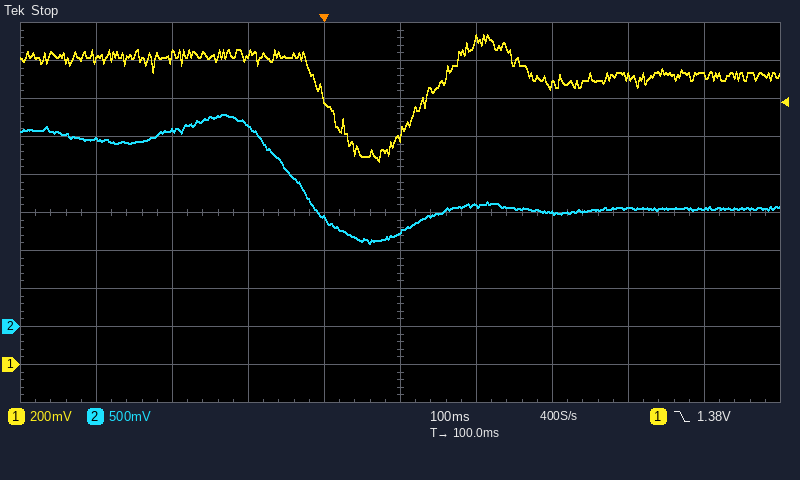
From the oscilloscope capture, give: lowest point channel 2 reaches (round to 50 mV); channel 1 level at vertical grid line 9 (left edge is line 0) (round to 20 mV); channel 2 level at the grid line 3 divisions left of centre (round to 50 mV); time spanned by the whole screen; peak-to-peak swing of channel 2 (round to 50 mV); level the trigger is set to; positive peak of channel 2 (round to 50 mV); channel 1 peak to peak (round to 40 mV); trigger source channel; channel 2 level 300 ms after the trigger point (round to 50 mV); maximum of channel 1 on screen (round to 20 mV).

1.10 V
1.52 V
2.60 V
1 s
1.70 V
1.38 V
2.80 V
680 mV
channel 1
1.50 V
1.74 V
